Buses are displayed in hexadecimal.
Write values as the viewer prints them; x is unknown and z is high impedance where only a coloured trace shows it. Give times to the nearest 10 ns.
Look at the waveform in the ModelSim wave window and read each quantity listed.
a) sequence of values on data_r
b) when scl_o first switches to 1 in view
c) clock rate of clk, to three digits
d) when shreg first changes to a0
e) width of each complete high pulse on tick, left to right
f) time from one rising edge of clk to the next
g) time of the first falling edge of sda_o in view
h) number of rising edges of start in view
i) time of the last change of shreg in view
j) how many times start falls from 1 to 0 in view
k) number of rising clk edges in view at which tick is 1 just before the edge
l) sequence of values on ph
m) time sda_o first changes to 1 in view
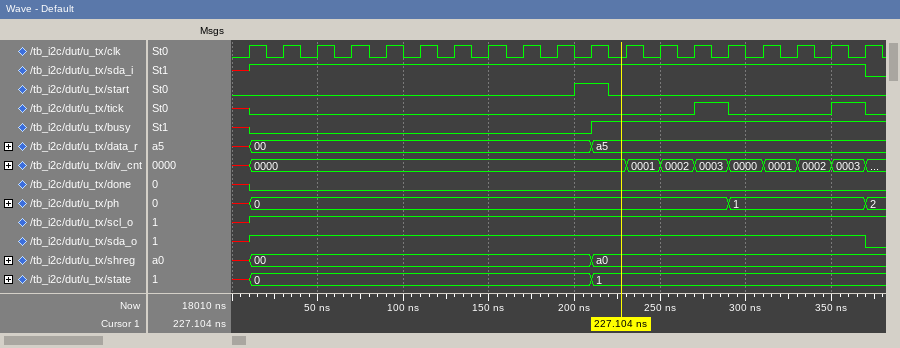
x, 00, a5
10 ns
50.0 MHz
210 ns
20 ns, 20 ns
20 ns
370 ns
1
210 ns
1
2
x, 0, 1, 2
10 ns
